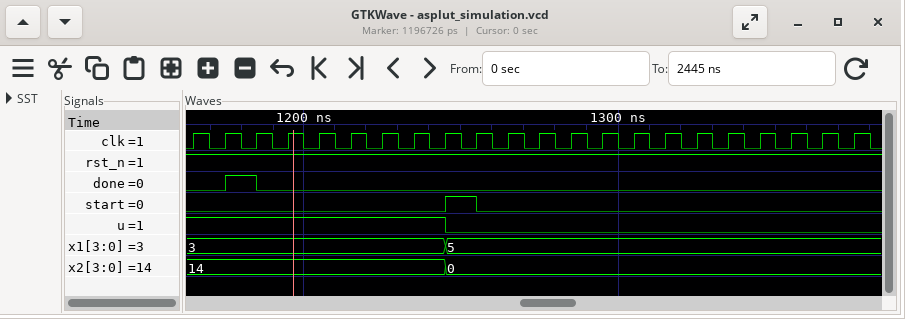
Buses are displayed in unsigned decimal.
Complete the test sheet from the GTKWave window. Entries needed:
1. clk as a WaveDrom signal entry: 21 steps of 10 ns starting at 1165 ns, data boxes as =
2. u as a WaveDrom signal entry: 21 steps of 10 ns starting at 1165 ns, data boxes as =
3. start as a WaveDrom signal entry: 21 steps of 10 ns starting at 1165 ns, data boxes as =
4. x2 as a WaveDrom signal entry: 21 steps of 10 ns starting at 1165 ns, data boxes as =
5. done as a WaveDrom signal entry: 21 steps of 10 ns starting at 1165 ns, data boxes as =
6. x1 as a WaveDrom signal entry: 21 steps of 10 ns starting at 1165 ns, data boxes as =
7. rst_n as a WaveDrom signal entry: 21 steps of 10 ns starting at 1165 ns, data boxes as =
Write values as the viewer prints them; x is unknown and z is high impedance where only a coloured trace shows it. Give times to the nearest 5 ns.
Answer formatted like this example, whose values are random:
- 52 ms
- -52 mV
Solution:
- {name: 'clk', wave: 'p....................'}
- {name: 'u', wave: '1.......0............'}
- {name: 'start', wave: '0.......10...........'}
- {name: 'x2', wave: '=.......=............', data: '14 0'}
- {name: 'done', wave: '010..................'}
- {name: 'x1', wave: '=.......=............', data: '3 5'}
- {name: 'rst_n', wave: '1....................'}
